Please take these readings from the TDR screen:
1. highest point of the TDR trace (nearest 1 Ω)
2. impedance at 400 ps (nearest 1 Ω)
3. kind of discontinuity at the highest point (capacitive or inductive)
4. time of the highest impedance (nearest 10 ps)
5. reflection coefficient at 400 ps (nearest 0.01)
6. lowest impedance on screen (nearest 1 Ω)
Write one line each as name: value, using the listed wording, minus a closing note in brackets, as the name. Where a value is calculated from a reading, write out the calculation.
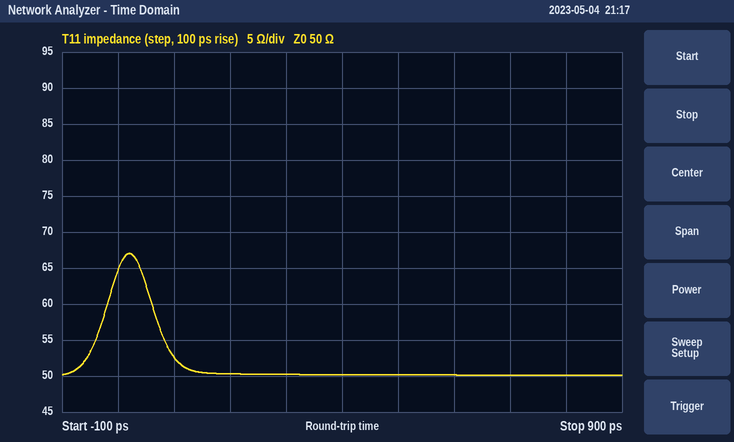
highest point of the TDR trace: 67 Ω
impedance at 400 ps: 50 Ω
kind of discontinuity at the highest point: inductive
time of the highest impedance: 20 ps
reflection coefficient at 400 ps: (50 − 50)/(50 + 50) ≈ 0.00
lowest impedance on screen: 50 Ω
